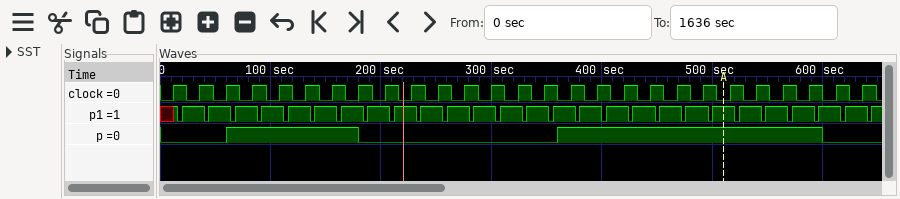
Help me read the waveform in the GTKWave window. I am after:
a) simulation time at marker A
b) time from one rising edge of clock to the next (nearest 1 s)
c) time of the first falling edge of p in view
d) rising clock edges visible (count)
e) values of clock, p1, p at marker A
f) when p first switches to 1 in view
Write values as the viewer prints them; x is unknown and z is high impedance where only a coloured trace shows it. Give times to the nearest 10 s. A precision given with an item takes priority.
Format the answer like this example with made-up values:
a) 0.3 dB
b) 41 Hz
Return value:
a) 510 s
b) 24 s
c) 180 s
d) 27
e) clock=0, p1=1, p=1
f) 60 s
